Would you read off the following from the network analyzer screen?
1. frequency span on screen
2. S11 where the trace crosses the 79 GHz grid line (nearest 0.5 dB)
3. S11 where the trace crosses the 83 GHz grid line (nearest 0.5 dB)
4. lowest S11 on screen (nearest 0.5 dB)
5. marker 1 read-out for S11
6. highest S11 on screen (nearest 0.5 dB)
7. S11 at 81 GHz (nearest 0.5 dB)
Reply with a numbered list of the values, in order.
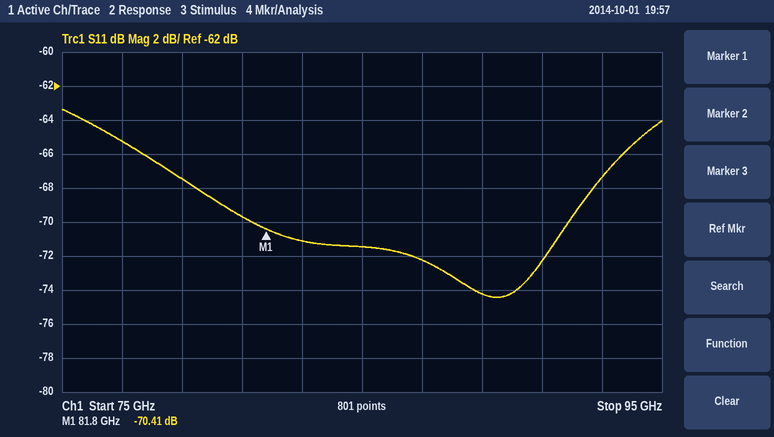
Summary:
1. 20 GHz
2. -67.5 dB
3. -71.0 dB
4. -74.5 dB
5. -70.41 dB
6. -63.5 dB
7. -69.5 dB
